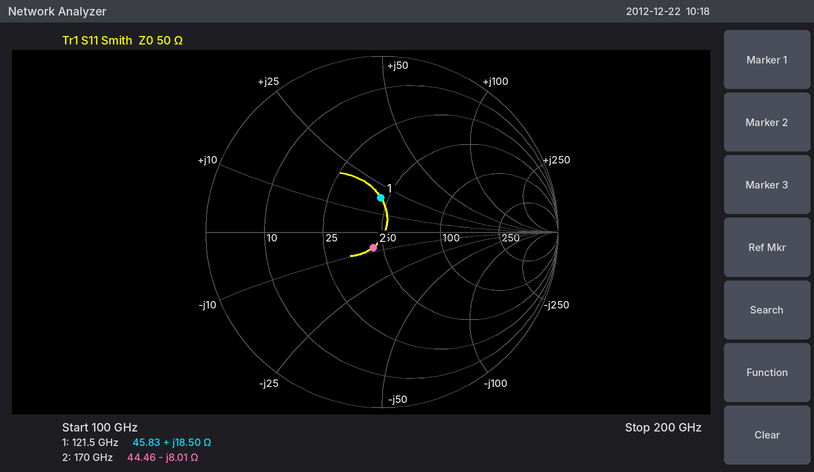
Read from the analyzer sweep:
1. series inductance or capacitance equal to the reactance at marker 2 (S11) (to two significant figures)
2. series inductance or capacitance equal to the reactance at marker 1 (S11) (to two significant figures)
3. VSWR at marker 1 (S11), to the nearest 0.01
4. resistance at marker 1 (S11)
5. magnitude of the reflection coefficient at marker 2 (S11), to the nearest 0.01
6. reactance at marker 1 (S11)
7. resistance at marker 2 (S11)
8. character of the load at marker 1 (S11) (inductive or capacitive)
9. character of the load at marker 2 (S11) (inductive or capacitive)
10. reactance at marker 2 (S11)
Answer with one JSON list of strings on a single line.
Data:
["120 fF", "24 pH", "1.48", "45.83 Ω", "0.10", "+18.50 Ω", "44.46 Ω", "inductive", "capacitive", "-8.01 Ω"]
